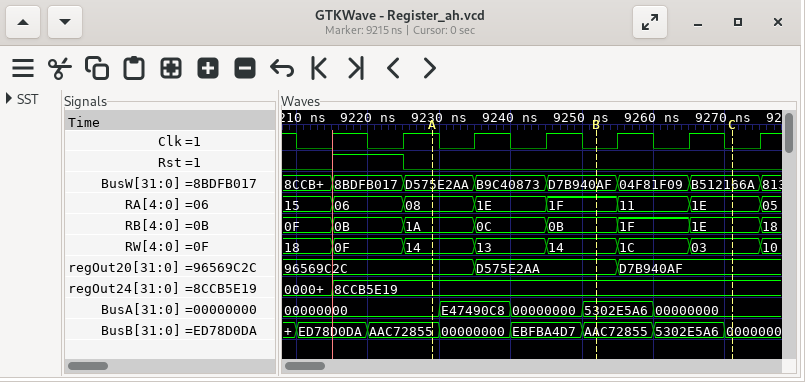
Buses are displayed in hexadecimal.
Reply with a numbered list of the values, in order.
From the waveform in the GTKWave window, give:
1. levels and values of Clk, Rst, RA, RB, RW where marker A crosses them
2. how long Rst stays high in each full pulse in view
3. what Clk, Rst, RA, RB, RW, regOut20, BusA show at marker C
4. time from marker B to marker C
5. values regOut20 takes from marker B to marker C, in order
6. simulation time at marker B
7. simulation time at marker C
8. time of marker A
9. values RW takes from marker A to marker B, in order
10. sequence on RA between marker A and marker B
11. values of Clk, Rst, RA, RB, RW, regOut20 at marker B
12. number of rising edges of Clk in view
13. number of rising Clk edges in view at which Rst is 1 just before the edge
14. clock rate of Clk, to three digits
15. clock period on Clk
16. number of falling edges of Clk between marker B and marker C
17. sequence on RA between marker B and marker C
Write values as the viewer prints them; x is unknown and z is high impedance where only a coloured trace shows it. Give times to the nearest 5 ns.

1. Clk=1, Rst=0, RA=08, RB=1A, RW=14
2. 10 ns
3. Clk=0, Rst=0, RA=1E, RB=1E, RW=03, regOut20=D7B940AF, BusA=00000000
4. 20 ns
5. D575E2AA, D7B940AF
6. 9250 ns
7. 9270 ns
8. 9230 ns
9. 14, 13, 14
10. 08, 1E, 1F
11. Clk=0, Rst=0, RA=1F, RB=0B, RW=14, regOut20=D575E2AA
12. 7
13. 1
14. 100 MHz
15. 10 ns
16. 2
17. 1F, 11, 1E
